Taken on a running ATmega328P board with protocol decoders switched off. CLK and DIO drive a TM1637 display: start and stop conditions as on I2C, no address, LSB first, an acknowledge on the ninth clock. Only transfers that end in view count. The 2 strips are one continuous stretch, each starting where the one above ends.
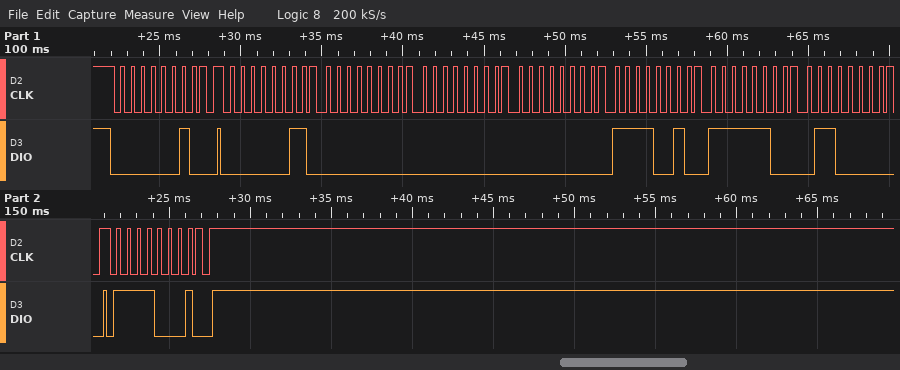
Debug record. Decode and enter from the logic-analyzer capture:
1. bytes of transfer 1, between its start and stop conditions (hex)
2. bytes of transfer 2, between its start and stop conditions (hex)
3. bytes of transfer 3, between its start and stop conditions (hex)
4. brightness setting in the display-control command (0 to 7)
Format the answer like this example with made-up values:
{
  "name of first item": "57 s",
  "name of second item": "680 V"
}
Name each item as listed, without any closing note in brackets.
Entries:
{
  "bytes of transfer 1, between its start and stop conditions": "40",
  "bytes of transfer 2, between its start and stop conditions": "C0 00 00 00 4F 3F 06",
  "bytes of transfer 3, between its start and stop conditions": "8F",
  "brightness setting in the display-control command": "7"
}
